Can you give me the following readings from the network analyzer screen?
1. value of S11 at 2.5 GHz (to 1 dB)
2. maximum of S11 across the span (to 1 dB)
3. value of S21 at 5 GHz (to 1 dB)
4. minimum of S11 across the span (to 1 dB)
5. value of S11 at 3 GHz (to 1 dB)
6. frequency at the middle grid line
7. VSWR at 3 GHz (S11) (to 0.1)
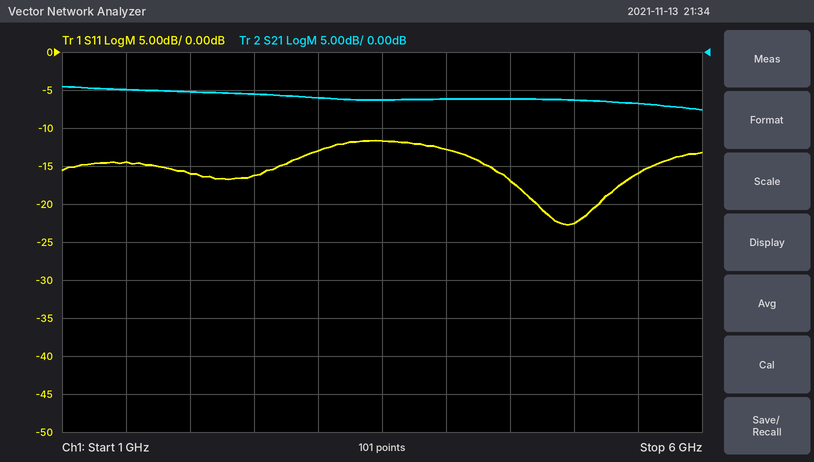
-16 dB
-12 dB
-6 dB
-23 dB
-13 dB
3.5 GHz
1.6
